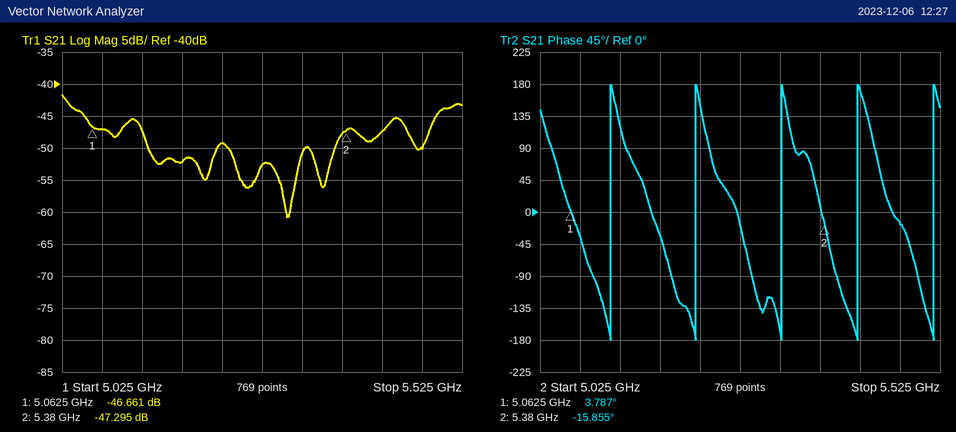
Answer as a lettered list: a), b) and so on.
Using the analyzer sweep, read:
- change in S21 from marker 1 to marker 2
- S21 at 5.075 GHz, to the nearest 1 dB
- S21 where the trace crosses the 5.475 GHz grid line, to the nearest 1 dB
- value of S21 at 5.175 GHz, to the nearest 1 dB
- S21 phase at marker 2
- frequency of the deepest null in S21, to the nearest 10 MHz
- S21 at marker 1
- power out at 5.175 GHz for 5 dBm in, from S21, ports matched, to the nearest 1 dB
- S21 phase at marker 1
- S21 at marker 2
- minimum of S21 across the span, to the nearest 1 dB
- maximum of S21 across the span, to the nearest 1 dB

a) -0.634 dB
b) -47 dB
c) -50 dB
d) -52 dB
e) -15.855°
f) 5.31 GHz
g) -46.661 dB
h) -47 dBm
i) 3.787°
j) -47.295 dB
k) -61 dB
l) -42 dB
